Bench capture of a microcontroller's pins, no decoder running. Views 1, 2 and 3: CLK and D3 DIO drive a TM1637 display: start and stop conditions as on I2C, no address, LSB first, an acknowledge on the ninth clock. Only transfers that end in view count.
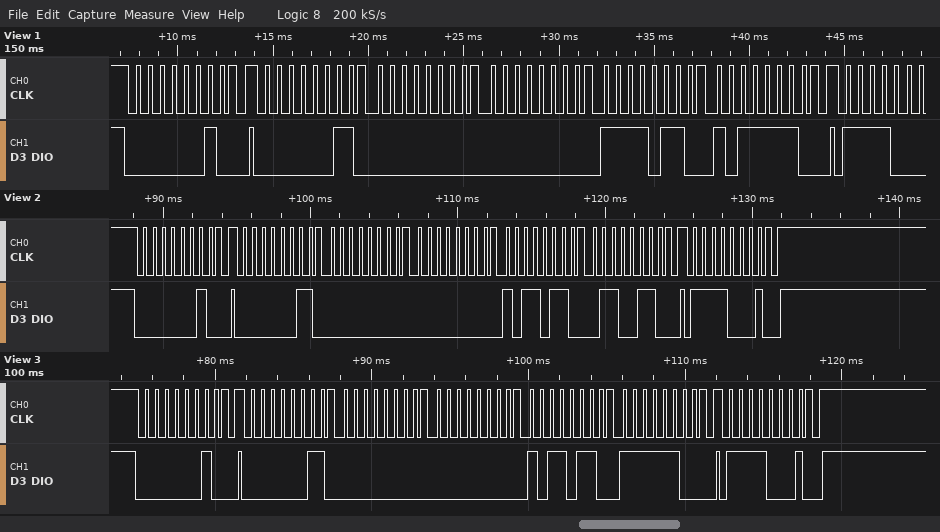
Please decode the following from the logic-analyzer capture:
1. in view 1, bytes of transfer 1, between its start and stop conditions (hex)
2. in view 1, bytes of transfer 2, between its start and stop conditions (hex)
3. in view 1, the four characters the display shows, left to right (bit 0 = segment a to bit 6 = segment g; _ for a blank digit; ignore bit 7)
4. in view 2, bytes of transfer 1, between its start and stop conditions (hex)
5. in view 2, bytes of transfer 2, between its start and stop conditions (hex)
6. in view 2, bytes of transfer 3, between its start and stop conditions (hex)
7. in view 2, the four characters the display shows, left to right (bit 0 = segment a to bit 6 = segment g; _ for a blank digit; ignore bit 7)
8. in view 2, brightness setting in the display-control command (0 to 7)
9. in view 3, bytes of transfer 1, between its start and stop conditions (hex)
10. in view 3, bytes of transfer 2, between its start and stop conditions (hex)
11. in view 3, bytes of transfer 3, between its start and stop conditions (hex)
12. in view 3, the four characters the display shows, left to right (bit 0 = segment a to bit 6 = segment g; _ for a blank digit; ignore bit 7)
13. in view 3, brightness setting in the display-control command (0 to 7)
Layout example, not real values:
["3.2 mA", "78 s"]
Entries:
["40", "C0 00 00 6F 7D", "__96", "40", "C0 00 00 6D 66", "8F", "__54", "7", "40", "C0 00 00 6D 3F", "8F", "__50", "7"]
